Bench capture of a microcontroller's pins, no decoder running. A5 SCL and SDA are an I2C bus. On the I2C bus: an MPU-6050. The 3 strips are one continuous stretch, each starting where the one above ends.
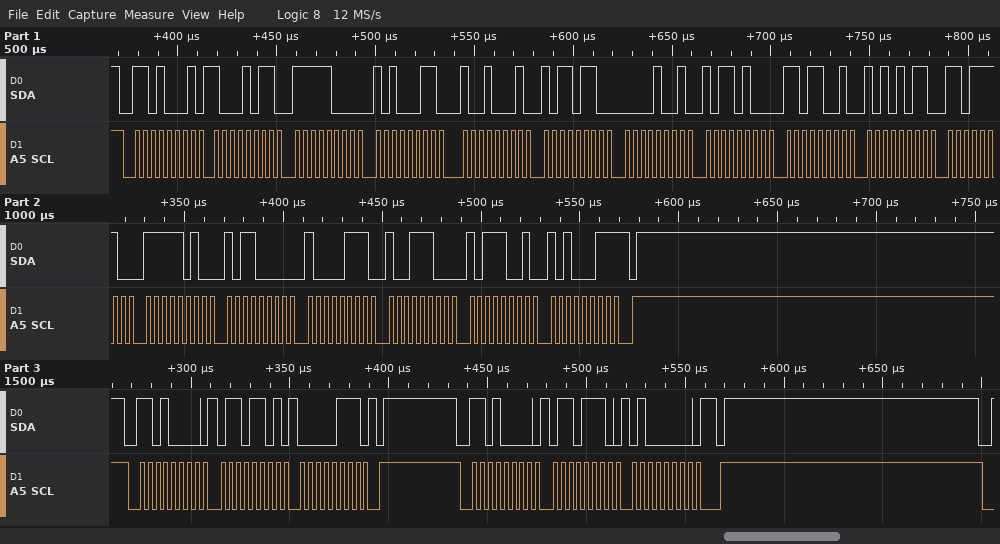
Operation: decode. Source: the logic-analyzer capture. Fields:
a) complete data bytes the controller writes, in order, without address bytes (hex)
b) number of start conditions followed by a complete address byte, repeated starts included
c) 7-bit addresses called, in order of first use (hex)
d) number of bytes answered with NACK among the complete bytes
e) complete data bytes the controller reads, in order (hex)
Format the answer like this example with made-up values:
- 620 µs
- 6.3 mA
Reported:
- 6D 07 6E 40
- 3
- 0x68
- 1
- 8B F8 A3 91 B6 09 B4 D9 AB DE FA B0 87 9C B9 A3
